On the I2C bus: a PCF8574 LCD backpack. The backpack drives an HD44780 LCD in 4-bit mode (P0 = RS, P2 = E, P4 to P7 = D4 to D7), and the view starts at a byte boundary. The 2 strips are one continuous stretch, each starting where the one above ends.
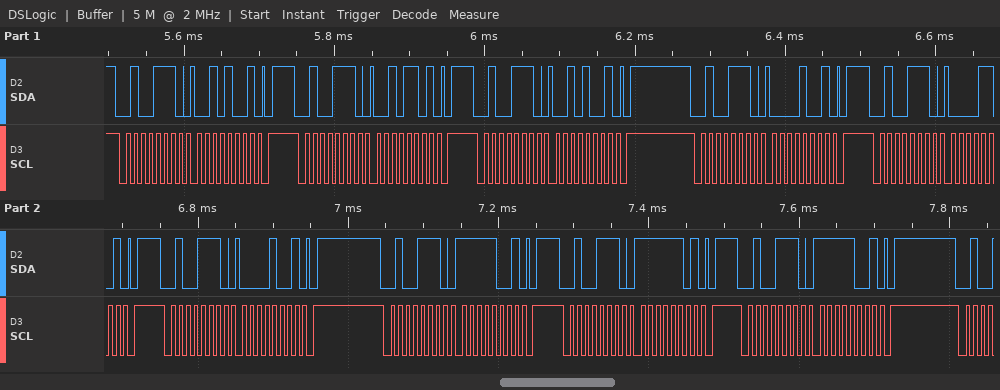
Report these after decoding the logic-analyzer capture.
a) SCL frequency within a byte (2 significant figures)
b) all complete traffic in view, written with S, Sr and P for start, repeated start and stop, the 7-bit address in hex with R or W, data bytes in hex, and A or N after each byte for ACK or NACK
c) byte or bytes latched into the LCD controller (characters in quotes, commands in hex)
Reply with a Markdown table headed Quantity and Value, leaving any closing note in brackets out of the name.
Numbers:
| Quantity | Value |
|---|---|
| SCL frequency within a byte | 100 kHz |
| all complete traffic in view, written with S, Sr and P for start, repeated start and stop, the 7-bit address in hex with R or W, data bytes in hex, and A or N after each byte for ACK or NACK | S 27W A 29 A P S 27W A 2D A P S 27W A 29 A P S 27W A 09 A P S 27W A 0D A P S 27W A 09 A P S 27W A F9 A P S 27W A FD A P S 27W A F9 A P |
| byte or bytes latched into the LCD controller | ' ' |
